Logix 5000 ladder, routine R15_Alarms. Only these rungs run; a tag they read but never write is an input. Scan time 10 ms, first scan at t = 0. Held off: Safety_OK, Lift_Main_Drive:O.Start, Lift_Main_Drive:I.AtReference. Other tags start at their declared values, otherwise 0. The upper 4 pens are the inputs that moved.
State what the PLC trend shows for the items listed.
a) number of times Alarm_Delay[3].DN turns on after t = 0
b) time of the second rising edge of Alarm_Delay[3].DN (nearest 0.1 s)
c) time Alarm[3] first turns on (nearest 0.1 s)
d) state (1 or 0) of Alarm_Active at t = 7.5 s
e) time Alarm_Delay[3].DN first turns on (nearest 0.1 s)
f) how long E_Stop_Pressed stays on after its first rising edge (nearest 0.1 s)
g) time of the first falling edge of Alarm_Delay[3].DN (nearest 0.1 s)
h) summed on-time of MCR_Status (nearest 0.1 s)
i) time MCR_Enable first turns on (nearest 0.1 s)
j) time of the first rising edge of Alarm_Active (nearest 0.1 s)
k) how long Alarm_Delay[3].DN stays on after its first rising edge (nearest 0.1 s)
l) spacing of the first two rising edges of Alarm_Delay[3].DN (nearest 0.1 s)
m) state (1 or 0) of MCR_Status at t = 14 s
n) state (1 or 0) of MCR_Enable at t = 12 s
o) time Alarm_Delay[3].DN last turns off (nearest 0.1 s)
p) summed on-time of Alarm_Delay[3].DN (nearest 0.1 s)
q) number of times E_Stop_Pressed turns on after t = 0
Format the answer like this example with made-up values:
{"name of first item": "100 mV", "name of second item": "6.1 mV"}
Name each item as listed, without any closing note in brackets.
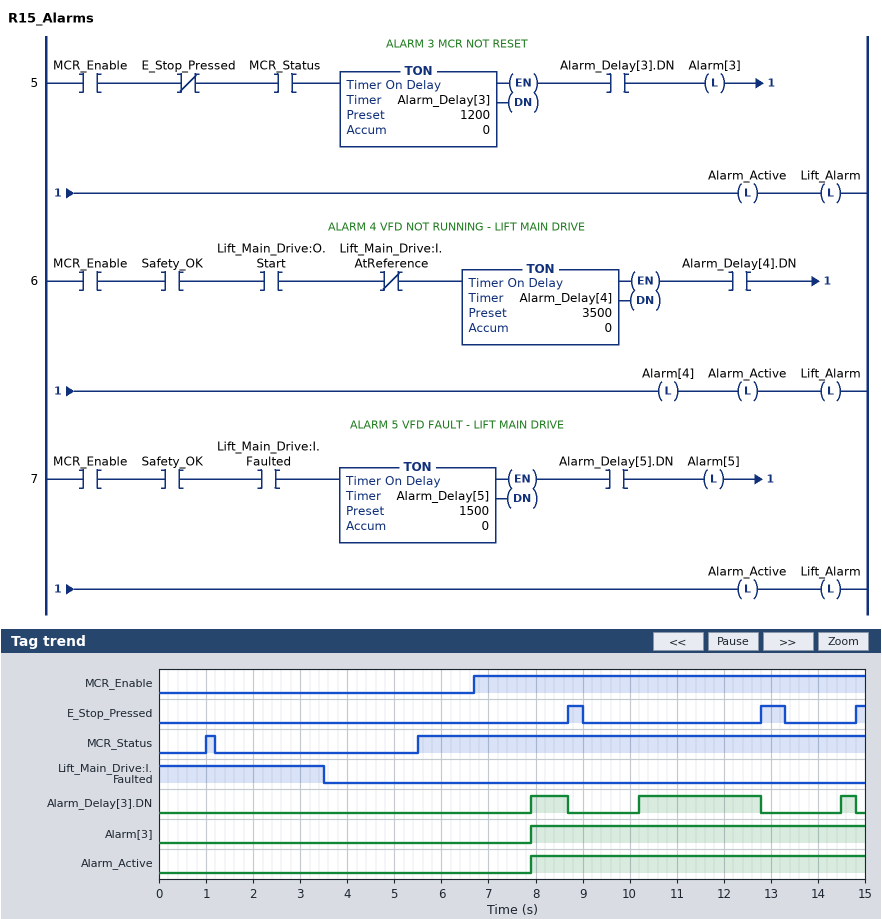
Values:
{"number of times Alarm_Delay[3].DN turns on after t = 0": "3", "time of the second rising edge of Alarm_Delay[3].DN": "10.2 s", "time Alarm[3] first turns on": "7.9 s", "state (1 or 0) of Alarm_Active at t = 7.5 s": "0", "time Alarm_Delay[3].DN first turns on": "7.9 s", "how long E_Stop_Pressed stays on after its first rising edge": "0.3 s", "time of the first falling edge of Alarm_Delay[3].DN": "8.7 s", "summed on-time of MCR_Status": "9.7 s", "time MCR_Enable first turns on": "6.7 s", "time of the first rising edge of Alarm_Active": "7.9 s", "how long Alarm_Delay[3].DN stays on after its first rising edge": "0.8 s", "spacing of the first two rising edges of Alarm_Delay[3].DN": "2.3 s", "state (1 or 0) of MCR_Status at t = 14 s": "1", "state (1 or 0) of MCR_Enable at t = 12 s": "1", "time Alarm_Delay[3].DN last turns off": "14.8 s", "summed on-time of Alarm_Delay[3].DN": "3.7 s", "number of times E_Stop_Pressed turns on after t = 0": "3"}
